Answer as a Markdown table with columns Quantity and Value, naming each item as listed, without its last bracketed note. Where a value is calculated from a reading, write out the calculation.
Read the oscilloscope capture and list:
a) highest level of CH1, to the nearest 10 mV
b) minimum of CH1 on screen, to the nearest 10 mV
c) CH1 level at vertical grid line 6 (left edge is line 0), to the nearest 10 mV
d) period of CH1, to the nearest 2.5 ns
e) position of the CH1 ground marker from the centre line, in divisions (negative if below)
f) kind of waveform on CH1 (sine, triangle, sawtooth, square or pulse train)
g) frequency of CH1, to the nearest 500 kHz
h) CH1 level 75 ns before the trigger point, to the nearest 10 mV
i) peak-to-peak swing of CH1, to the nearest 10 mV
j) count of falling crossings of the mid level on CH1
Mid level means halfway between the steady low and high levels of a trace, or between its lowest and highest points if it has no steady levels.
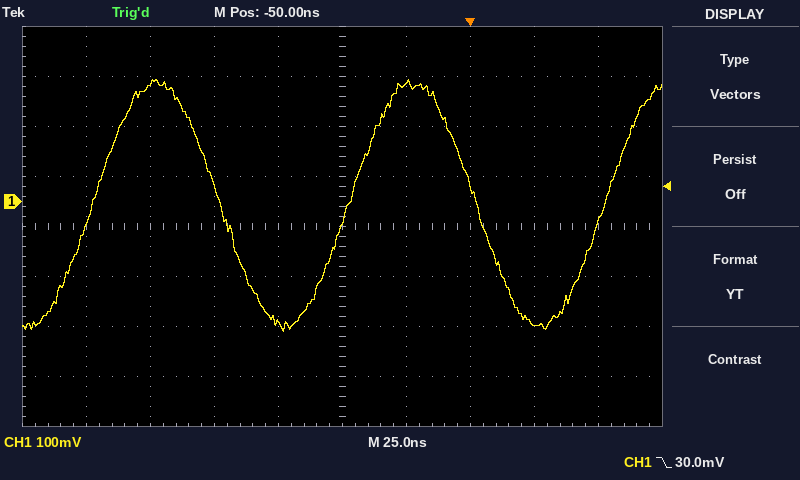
| Quantity | Value |
|---|---|
| highest level of CH1, to the nearest 10 mV | 240 mV |
| minimum of CH1 on screen, to the nearest 10 mV | -260 mV |
| CH1 level at vertical grid line 6 (left edge is line 0), to the nearest 10 mV | 240 mV |
| period of CH1, to the nearest 2.5 ns | 100.0 ns |
| position of the CH1 ground marker from the centre line, in divisions | +0.5 div |
| kind of waveform on CH1 | sine |
| frequency of CH1, to the nearest 500 kHz | 1 / 100.0 ns ≈ 10.0 MHz |
| CH1 level 75 ns before the trigger point, to the nearest 10 mV | -240 mV |
| peak-to-peak swing of CH1, to the nearest 10 mV | 240 mV − (-260 mV) = 500 mV |
| count of falling crossings of the mid level on CH1 | 2 |
